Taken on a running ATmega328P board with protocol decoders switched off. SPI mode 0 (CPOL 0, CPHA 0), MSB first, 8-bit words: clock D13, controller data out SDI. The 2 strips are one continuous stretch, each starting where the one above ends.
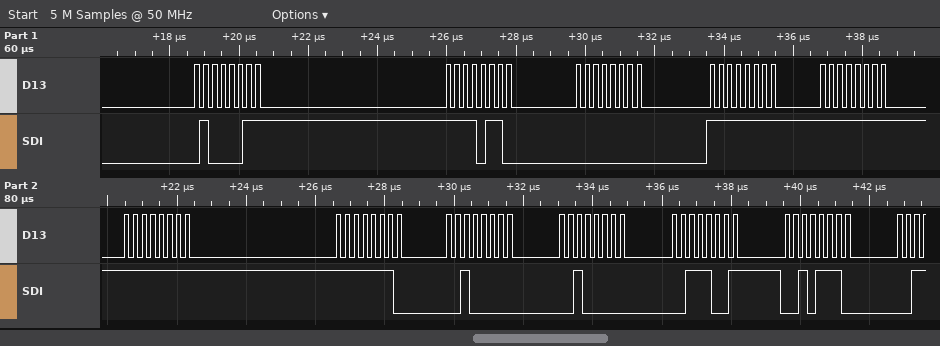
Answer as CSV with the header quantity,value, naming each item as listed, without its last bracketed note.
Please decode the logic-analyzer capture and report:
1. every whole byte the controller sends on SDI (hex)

quantity,value
every whole byte the controller sends on SDI,43 F6 00 FF FF FF FE 20 20 39 2E
